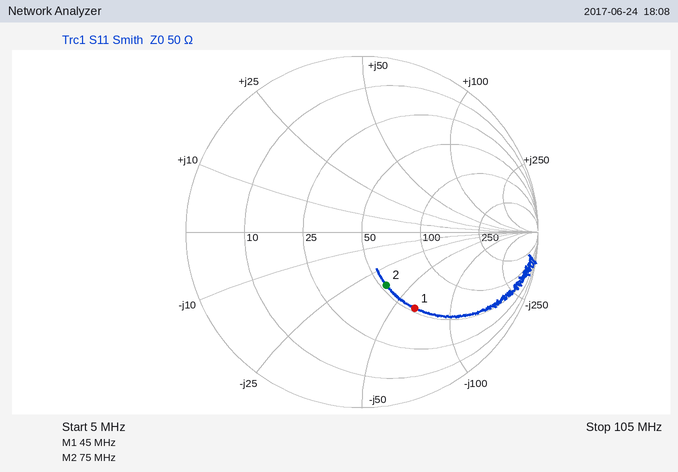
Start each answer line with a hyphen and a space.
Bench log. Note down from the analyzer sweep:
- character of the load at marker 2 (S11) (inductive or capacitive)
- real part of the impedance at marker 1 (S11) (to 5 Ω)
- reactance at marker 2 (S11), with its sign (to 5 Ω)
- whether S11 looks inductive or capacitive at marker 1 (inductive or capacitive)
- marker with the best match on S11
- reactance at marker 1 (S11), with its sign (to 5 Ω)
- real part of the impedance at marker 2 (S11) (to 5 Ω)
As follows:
- capacitive
- 55 Ω
- -35 Ω
- capacitive
- marker 2
- -65 Ω
- 55 Ω
